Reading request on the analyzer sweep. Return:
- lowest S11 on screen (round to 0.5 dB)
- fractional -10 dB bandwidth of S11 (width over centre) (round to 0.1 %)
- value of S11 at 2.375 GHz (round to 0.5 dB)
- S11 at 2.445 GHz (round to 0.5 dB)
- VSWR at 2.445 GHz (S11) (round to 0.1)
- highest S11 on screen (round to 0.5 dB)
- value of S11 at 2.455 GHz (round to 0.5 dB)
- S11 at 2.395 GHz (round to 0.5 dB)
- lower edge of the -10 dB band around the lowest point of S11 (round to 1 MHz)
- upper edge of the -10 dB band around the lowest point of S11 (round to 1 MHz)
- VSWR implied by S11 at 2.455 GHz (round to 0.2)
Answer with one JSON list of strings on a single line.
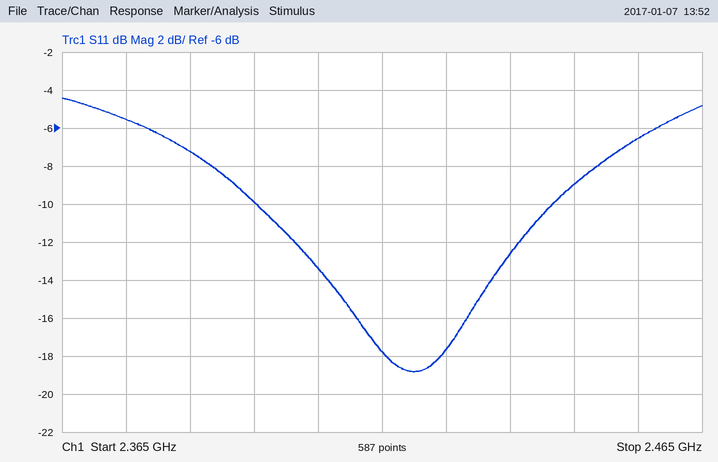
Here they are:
["-19.0 dB", "1.9 %", "-5.5 dB", "-9.0 dB", "2.1", "-4.5 dB", "-6.5 dB", "-10.0 dB", "2.395 GHz", "2.442 GHz", "2.8"]
